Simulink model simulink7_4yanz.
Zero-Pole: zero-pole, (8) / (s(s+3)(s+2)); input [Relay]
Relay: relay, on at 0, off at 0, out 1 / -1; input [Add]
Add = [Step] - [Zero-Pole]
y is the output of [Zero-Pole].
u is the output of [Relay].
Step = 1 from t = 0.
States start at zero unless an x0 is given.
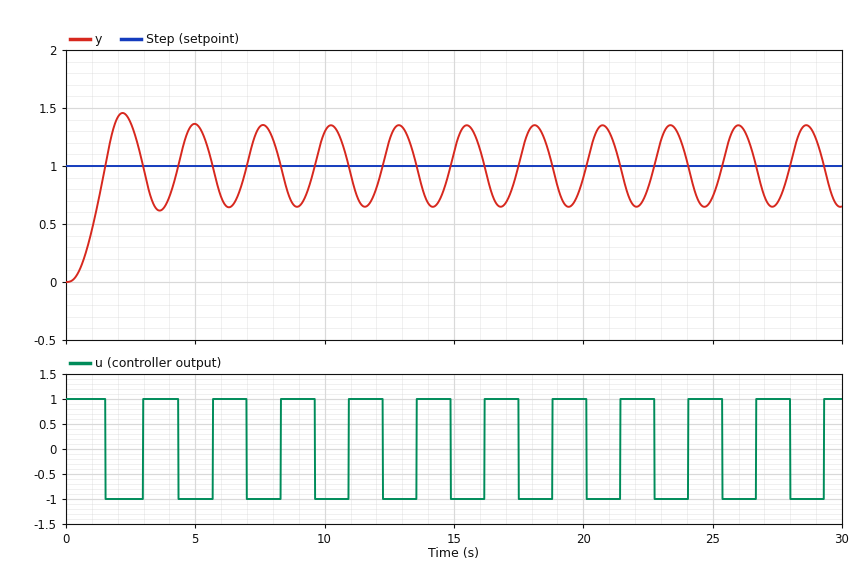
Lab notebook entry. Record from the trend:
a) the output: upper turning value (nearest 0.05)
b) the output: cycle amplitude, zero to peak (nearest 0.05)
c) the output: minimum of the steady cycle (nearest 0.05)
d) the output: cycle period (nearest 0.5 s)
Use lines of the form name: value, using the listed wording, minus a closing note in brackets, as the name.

the output: upper turning value: 1.35
the output: cycle amplitude, zero to peak: 0.35
the output: minimum of the steady cycle: 0.65
the output: cycle period: 2.5 s
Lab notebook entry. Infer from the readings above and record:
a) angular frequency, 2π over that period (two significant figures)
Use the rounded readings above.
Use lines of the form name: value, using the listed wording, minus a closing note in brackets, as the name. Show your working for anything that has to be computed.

angular frequency, 2π over that period: 2π / 2.5 = 2.5 rad/s
